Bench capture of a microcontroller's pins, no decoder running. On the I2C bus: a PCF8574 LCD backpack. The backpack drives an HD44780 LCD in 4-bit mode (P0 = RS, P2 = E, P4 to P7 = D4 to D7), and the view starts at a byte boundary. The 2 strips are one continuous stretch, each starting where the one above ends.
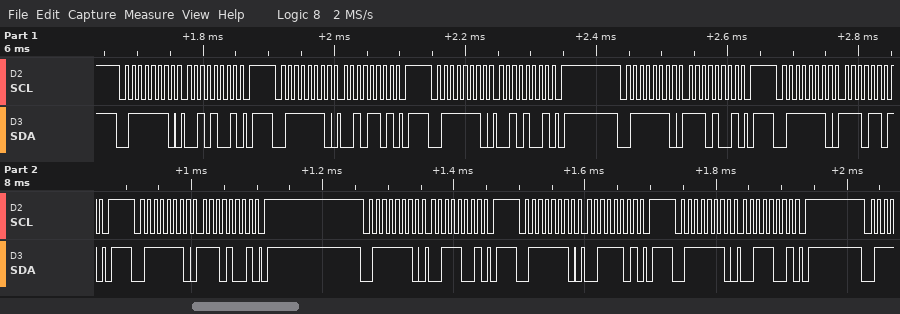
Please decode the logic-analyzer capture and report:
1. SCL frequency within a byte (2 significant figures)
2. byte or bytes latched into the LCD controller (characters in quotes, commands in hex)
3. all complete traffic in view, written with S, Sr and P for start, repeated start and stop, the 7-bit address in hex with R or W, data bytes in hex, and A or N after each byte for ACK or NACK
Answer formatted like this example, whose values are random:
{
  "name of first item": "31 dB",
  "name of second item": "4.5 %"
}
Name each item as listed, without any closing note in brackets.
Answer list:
{
  "SCL frequency within a byte": "100 kHz",
  "byte or bytes latched into the LCD controller": "'.'",
  "all complete traffic in view, written with S, Sr and P for start, repeated start and stop, the 7-bit address in hex with R or W, data bytes in hex, and A or N after each byte for ACK or NACK": "S 3FW A 29 A P S 3FW A 2D A P S 3FW A 29 A P S 3FW A E9 A P S 3FW A ED A P S 3FW A E9 A P S 3FW A 39 A P S 3FW A 3D A P S 3FW A 39 A P"
}
